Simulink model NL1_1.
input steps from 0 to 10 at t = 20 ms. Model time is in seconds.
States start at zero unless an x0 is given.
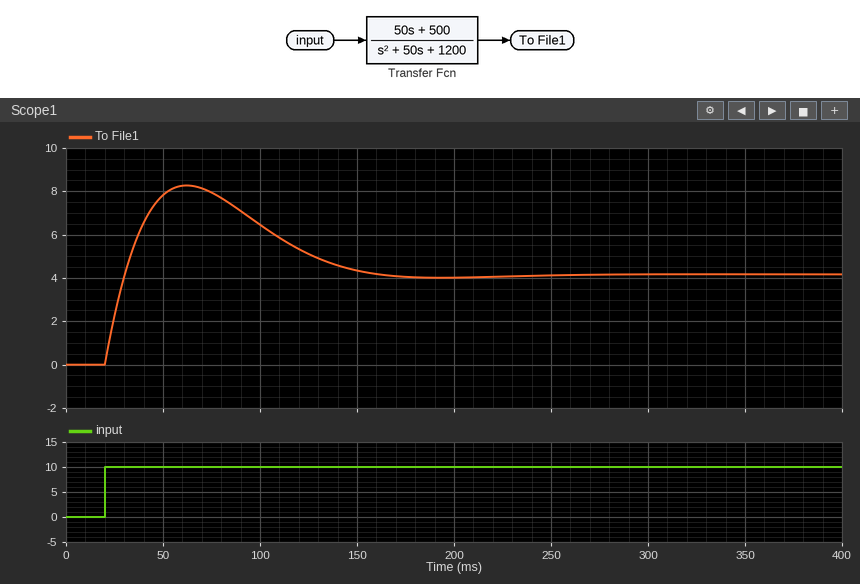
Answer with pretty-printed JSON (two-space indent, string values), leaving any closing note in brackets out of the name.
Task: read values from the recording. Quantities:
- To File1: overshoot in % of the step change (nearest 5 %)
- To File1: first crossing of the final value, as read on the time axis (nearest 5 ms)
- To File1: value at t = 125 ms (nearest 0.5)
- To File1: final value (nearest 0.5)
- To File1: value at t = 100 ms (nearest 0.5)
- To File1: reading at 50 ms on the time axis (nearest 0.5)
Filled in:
{
  "To File1: overshoot in % of the step change": "100 %",
  "To File1: first crossing of the final value, as read on the time axis": "30 ms",
  "To File1: value at t = 125 ms": "5.0",
  "To File1: final value": "4.0",
  "To File1: value at t = 100 ms": "6.5",
  "To File1: reading at 50 ms on the time axis": "8.0"
}
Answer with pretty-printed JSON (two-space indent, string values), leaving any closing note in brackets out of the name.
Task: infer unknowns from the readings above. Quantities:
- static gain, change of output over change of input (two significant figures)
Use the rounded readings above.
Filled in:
{
  "static gain, change of output over change of input": "0.40"
}
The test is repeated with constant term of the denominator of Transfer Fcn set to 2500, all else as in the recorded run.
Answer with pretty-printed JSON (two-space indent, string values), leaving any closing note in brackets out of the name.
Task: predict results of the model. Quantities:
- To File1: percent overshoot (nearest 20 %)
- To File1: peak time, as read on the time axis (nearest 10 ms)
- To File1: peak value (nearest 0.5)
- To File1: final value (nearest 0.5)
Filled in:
{
  "To File1: percent overshoot": "220 %",
  "To File1: peak time, as read on the time axis": "50 ms",
  "To File1: peak value": "6.5",
  "To File1: final value": "2.0"
}
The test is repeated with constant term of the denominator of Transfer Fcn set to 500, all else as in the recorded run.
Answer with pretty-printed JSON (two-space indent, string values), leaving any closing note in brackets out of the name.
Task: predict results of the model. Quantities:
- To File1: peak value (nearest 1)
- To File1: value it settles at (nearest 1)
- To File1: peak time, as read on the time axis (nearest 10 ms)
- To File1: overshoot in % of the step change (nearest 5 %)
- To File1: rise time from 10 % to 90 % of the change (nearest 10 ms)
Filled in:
{
  "To File1: peak value": "11",
  "To File1: value it settles at": "10",
  "To File1: peak time, as read on the time axis": "110 ms",
  "To File1: overshoot in % of the step change": "10 %",
  "To File1: rise time from 10 % to 90 % of the change": "30 ms"
}
